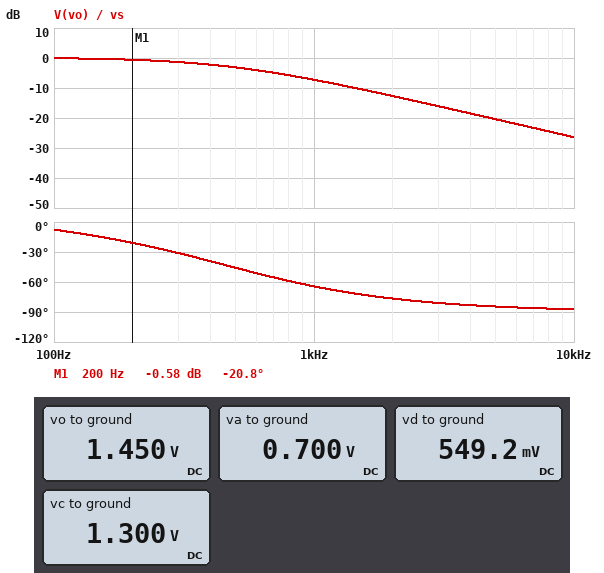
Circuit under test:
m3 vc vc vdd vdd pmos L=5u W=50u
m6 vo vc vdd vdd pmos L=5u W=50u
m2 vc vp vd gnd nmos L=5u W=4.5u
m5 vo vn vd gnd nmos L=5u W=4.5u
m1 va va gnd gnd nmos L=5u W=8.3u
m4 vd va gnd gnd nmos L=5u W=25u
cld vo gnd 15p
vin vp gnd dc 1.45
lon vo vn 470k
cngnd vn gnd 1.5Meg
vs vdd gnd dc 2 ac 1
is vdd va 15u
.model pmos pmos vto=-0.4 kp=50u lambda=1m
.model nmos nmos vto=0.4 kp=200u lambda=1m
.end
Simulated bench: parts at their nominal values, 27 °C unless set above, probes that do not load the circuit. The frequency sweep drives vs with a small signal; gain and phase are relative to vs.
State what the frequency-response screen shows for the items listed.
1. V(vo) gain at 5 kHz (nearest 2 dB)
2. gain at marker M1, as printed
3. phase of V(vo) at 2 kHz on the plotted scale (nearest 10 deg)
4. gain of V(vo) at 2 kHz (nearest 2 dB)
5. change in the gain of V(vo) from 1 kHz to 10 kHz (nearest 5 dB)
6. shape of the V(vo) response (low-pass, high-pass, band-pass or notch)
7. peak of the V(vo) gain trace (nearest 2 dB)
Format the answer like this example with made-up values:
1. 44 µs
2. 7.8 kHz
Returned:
1. -20 dB
2. -0.58 dB
3. -80 deg
4. -12 dB
5. -20 dB
6. low-pass
7. 0 dB
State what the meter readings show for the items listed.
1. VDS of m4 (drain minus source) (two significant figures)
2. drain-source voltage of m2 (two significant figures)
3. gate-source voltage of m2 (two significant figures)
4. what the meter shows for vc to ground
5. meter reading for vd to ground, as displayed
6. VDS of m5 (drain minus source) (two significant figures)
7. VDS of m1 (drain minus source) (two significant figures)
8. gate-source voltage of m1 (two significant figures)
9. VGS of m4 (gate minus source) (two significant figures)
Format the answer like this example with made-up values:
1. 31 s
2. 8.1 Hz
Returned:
1. 550 mV
2. 750 mV
3. 900 mV
4. 1.300 V
5. 549.2 mV
6. 900 mV
7. 700 mV
8. 700 mV
9. 700 mV
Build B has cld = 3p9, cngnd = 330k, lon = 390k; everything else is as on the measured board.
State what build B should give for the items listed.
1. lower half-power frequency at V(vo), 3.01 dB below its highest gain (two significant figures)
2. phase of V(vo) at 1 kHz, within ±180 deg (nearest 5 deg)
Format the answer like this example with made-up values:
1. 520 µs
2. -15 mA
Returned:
1. 9.0 Hz
2. -30 deg
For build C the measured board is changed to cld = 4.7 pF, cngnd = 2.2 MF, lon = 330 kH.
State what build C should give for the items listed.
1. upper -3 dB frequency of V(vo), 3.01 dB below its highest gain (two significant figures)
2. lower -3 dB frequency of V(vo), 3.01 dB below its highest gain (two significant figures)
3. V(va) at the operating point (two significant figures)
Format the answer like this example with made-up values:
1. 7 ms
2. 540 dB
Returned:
1. 1.5 kHz
2. 11 Hz
3. 700 mV
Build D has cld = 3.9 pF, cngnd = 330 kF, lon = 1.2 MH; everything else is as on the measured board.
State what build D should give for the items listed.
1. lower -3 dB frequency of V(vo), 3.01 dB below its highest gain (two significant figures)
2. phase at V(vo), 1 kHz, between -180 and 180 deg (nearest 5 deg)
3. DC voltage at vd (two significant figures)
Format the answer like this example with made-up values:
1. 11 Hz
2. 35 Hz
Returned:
1. 2.9 Hz
2. -30 deg
3. 550 mV
